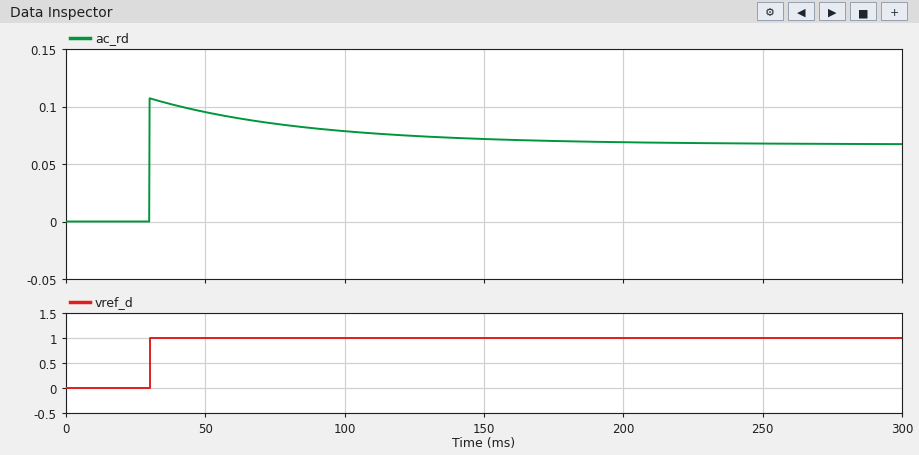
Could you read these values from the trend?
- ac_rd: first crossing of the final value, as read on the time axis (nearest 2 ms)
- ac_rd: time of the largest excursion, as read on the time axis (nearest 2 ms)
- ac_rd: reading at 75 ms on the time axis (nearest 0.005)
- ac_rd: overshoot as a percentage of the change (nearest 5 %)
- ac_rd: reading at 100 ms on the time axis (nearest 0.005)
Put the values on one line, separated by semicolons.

30 ms; 30 ms; 0.085; 60 %; 0.080
